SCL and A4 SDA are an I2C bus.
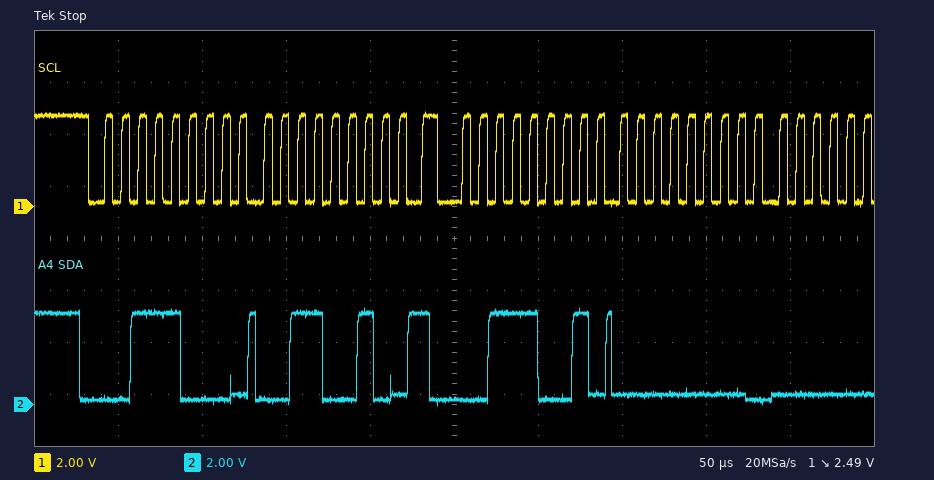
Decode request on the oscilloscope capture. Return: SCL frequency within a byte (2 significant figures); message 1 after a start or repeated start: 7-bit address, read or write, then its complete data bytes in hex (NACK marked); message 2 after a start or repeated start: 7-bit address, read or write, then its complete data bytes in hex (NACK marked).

100 kHz
0x1C write: 32
0x1C read: 00
